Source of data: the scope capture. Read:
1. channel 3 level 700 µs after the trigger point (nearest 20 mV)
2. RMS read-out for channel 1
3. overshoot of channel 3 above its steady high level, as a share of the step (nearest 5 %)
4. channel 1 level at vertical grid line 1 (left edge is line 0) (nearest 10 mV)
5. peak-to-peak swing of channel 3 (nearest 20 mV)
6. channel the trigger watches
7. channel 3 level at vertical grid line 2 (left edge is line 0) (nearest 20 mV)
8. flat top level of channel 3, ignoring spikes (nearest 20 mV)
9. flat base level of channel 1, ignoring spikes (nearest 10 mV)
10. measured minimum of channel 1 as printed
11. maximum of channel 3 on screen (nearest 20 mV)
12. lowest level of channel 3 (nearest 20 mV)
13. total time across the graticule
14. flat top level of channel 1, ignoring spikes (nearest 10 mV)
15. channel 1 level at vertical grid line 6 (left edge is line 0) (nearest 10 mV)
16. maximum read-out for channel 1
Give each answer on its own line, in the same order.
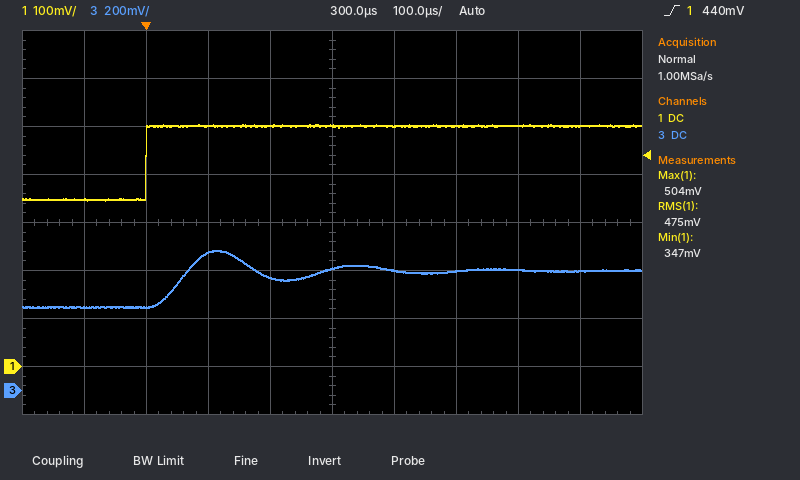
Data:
500 mV
475 mV
55 %
350 mV
240 mV
channel 1
340 mV
500 mV
350 mV
347 mV
580 mV
340 mV
1 ms
500 mV
500 mV
504 mV
